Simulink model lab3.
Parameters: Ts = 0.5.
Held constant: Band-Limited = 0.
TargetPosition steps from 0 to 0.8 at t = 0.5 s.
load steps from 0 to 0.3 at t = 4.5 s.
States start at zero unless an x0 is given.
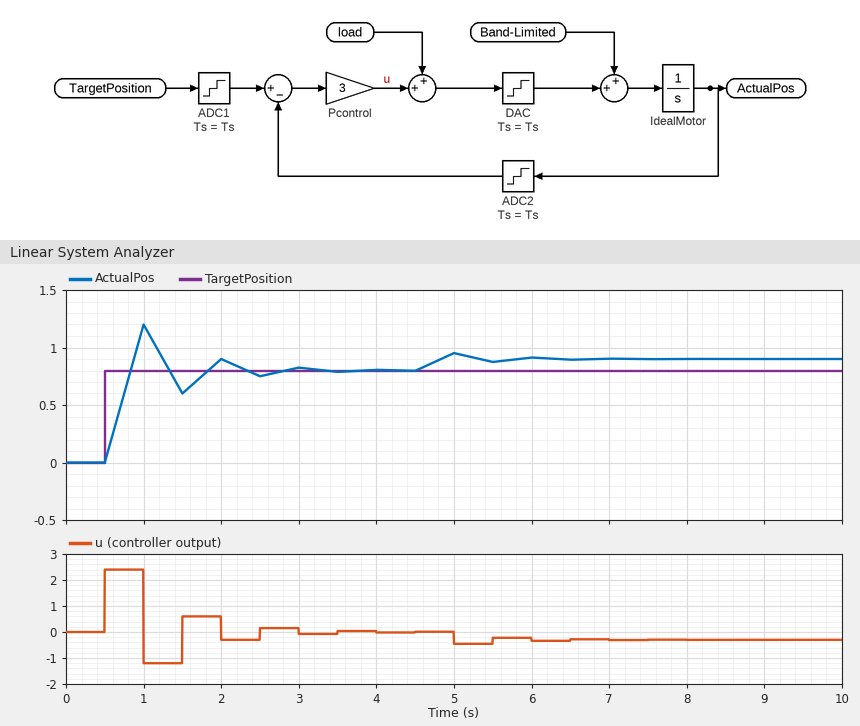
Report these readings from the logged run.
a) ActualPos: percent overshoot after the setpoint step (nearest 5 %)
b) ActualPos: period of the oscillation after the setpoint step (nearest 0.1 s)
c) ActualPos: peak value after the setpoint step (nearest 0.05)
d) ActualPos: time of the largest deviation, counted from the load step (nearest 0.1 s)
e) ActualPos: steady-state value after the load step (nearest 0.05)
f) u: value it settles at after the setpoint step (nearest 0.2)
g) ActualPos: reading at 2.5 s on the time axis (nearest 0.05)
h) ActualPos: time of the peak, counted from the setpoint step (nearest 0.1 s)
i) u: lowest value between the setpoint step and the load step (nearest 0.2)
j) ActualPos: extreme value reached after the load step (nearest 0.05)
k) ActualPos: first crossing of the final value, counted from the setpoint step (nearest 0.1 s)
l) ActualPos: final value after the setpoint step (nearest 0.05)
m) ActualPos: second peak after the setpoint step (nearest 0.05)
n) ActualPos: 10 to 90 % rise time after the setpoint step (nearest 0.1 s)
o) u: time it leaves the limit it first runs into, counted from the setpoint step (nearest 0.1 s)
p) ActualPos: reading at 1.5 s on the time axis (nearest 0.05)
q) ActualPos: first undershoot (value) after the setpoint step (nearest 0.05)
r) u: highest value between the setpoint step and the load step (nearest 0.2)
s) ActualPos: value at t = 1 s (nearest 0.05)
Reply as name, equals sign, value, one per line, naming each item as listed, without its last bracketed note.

ActualPos: percent overshoot after the setpoint step = 50 %
ActualPos: period of the oscillation after the setpoint step = 1.0 s
ActualPos: peak value after the setpoint step = 1.20
ActualPos: time of the largest deviation, counted from the load step = 0.5 s
ActualPos: steady-state value after the load step = 0.90
u: value it settles at after the setpoint step = 0.0
ActualPos: reading at 2.5 s on the time axis = 0.75
ActualPos: time of the peak, counted from the setpoint step = 0.5 s
u: lowest value between the setpoint step and the load step = -1.2
ActualPos: extreme value reached after the load step = 0.95
ActualPos: first crossing of the final value, counted from the setpoint step = 0.3 s
ActualPos: final value after the setpoint step = 0.80
ActualPos: second peak after the setpoint step = 0.90
ActualPos: 10 to 90 % rise time after the setpoint step = 0.3 s
u: time it leaves the limit it first runs into, counted from the setpoint step = 0.5 s
ActualPos: reading at 1.5 s on the time axis = 0.60
ActualPos: first undershoot (value) after the setpoint step = 0.60
u: highest value between the setpoint step and the load step = 2.4
ActualPos: value at t = 1 s = 1.20
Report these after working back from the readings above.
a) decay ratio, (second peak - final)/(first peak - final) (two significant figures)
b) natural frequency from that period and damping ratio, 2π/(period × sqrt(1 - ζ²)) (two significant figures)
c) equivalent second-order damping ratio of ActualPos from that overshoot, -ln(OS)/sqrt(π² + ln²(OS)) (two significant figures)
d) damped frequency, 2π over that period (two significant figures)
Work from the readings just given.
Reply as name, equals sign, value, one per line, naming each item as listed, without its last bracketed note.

decay ratio, (second peak - final)/(first peak - final) = 0.25
natural frequency from that period and damping ratio, 2π/(period × sqrt(1 - ζ²)) = 6.4 rad/s
equivalent second-order damping ratio of ActualPos from that overshoot, -ln(OS)/sqrt(π² + ln²(OS)) = 0.22
damped frequency, 2π over that period = 6.3 rad/s
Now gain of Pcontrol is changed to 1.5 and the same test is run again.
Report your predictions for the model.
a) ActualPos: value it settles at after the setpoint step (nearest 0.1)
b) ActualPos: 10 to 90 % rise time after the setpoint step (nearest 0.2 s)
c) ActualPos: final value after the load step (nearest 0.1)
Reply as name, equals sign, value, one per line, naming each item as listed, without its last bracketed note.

ActualPos: value it settles at after the setpoint step = 0.8
ActualPos: 10 to 90 % rise time after the setpoint step = 0.8 s
ActualPos: final value after the load step = 1.0
